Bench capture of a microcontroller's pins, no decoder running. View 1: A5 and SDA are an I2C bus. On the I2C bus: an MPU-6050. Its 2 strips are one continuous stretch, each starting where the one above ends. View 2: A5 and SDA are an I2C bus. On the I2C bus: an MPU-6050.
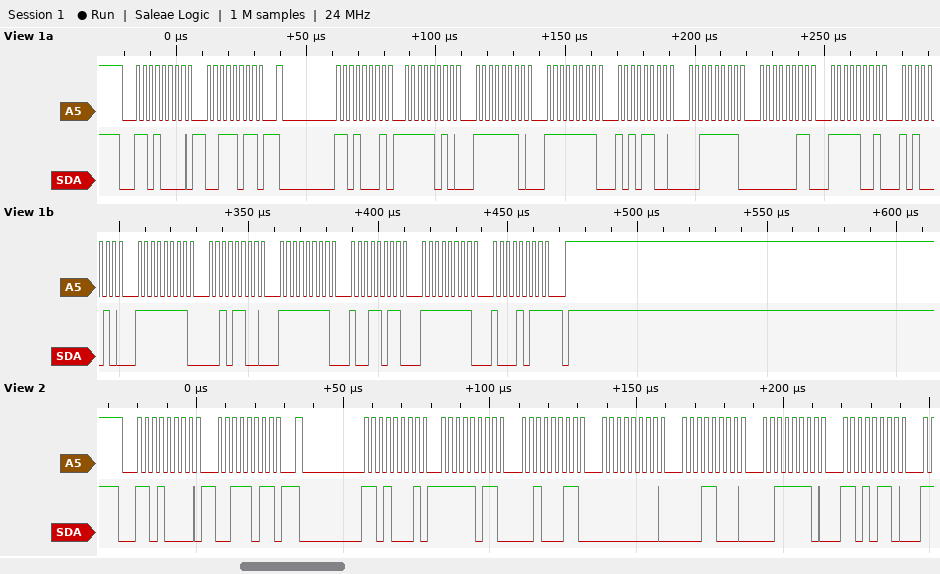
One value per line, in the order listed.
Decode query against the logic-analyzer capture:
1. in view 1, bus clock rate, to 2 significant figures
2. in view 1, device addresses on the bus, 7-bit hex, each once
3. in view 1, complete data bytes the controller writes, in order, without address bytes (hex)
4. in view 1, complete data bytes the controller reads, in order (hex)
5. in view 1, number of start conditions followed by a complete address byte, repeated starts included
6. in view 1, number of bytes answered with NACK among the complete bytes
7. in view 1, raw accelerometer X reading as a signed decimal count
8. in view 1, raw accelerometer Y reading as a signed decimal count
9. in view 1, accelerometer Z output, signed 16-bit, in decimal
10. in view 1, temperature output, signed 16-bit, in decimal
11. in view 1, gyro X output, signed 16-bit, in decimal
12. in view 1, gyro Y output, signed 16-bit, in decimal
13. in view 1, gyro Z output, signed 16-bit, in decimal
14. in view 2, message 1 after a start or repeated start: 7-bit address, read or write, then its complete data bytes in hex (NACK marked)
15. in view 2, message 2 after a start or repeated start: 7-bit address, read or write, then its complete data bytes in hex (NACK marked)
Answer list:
400 kHz
0x68
3B
FA FE FF AC 3F 03 F9 A2 FF 2C FF 9B FF 8B
2
1
-1282
-84
16131
-1630
-212
-101
-117
0x68 write: 3B
0x68 read: FB 23 00 18 3E D6
